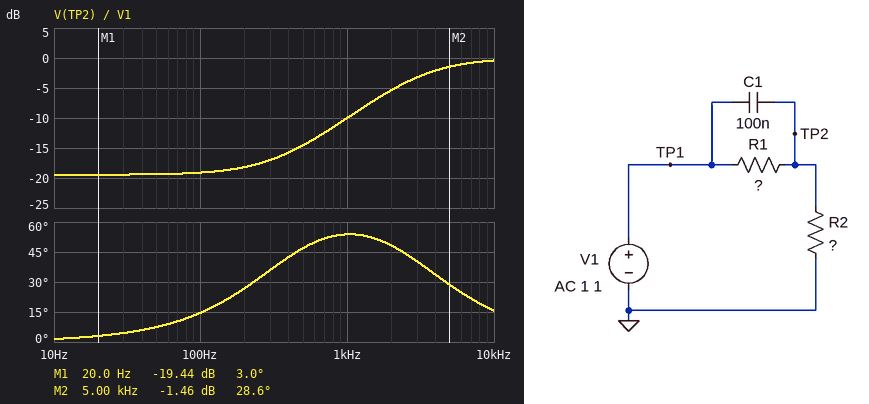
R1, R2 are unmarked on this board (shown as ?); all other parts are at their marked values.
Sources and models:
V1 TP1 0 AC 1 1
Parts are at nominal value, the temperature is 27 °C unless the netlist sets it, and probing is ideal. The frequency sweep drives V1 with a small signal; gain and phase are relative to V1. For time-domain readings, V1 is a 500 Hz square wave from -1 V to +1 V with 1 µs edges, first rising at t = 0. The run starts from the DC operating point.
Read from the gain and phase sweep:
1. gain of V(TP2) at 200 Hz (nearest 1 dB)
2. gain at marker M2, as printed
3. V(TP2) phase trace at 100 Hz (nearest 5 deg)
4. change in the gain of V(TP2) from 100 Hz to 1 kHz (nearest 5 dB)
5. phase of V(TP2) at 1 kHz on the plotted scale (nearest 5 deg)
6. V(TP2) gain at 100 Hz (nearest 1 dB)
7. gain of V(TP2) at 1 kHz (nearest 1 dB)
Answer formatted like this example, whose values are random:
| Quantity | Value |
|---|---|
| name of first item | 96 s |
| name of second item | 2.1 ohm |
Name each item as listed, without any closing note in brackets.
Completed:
| Quantity | Value |
|---|---|
| gain of V(TP2) at 200 Hz | -18 dB |
| gain at marker M2, as printed | -1.46 dB |
| V(TP2) phase trace at 100 Hz | 15 deg |
| change in the gain of V(TP2) from 100 Hz to 1 kHz | 10 dB |
| phase of V(TP2) at 1 kHz on the plotted scale | 55 deg |
| V(TP2) gain at 100 Hz | -19 dB |
| gain of V(TP2) at 1 kHz | -10 dB |
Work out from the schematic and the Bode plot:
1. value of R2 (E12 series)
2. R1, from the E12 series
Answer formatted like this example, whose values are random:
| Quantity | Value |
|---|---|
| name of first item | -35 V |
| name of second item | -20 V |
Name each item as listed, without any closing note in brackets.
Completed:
| Quantity | Value |
|---|---|
| value of R2 | 560 Ω |
| R1, from the E12 series | 4.7 kΩ |
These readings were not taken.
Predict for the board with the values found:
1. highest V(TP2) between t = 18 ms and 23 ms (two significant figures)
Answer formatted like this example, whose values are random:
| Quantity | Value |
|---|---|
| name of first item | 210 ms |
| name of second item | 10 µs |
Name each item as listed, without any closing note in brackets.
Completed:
| Quantity | Value |
|---|---|
| highest V(TP2) between t = 18 ms and 23 ms | 1.9 V |
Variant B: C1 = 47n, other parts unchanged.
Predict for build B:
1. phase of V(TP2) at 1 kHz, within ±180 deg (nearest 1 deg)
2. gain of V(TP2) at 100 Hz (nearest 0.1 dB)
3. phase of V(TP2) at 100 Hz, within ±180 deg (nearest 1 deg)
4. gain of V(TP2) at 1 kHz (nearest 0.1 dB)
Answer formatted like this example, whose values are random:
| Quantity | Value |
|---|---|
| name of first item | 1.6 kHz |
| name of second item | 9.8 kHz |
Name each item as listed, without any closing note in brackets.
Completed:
| Quantity | Value |
|---|---|
| phase of V(TP2) at 1 kHz, within ±180 deg | 46 deg |
| gain of V(TP2) at 100 Hz | -19.4 dB |
| phase of V(TP2) at 100 Hz, within ±180 deg | 7 deg |
| gain of V(TP2) at 1 kHz | -14.9 dB |
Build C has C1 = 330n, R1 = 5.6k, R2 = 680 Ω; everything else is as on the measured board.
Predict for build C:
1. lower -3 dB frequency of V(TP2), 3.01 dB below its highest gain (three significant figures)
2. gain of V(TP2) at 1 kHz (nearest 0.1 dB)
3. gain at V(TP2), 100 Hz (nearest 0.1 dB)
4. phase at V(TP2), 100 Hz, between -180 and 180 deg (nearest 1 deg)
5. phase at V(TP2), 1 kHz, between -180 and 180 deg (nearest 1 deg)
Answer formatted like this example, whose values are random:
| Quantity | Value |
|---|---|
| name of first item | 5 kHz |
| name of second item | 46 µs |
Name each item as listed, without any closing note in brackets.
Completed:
| Quantity | Value |
|---|---|
| lower -3 dB frequency of V(TP2), 3.01 dB below its highest gain | 786 Hz |
| gain of V(TP2) at 1 kHz | -2.1 dB |
| gain at V(TP2), 100 Hz | -15.7 dB |
| phase at V(TP2), 100 Hz, between -180 and 180 deg | 42 deg |
| phase at V(TP2), 1 kHz, between -180 and 180 deg | 34 deg |
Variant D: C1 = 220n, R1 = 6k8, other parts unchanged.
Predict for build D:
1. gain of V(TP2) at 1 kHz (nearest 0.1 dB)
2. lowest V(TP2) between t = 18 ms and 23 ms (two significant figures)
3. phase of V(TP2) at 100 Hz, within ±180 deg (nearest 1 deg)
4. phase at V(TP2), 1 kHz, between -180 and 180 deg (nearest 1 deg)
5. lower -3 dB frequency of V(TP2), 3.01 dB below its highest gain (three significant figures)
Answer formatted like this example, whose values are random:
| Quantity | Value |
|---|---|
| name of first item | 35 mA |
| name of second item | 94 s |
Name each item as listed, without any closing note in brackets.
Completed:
| Quantity | Value |
|---|---|
| gain of V(TP2) at 1 kHz | -4.7 dB |
| lowest V(TP2) between t = 18 ms and 23 ms | -1.9 V |
| phase of V(TP2) at 100 Hz, within ±180 deg | 39 deg |
| phase at V(TP2), 1 kHz, between -180 and 180 deg | 48 deg |
| lower -3 dB frequency of V(TP2), 3.01 dB below its highest gain | 1.39 kHz |
